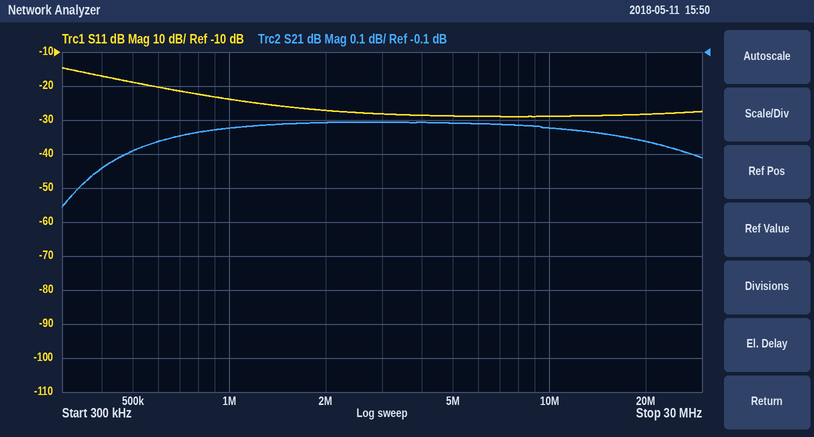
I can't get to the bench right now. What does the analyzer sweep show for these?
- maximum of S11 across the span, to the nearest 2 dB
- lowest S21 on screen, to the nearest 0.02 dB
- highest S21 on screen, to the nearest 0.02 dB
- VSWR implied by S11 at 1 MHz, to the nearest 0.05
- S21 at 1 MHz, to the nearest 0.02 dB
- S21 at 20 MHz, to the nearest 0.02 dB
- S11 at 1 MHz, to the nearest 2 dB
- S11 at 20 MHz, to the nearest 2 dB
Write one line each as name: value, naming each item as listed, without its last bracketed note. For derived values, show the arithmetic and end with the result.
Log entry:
maximum of S11 across the span, to the nearest 2 dB: -14 dB
lowest S21 on screen, to the nearest 0.02 dB: -0.56 dB
highest S21 on screen, to the nearest 0.02 dB: -0.30 dB
VSWR implied by S11 at 1 MHz, to the nearest 0.05: |Γ| = 10^(-24/20) = 0.0631; VSWR = (1 + 0.0631)/(1 − 0.0631) ≈ 1.13, so 1.15 to the nearest 0.05
S21 at 1 MHz, to the nearest 0.02 dB: -0.32 dB
S21 at 20 MHz, to the nearest 0.02 dB: -0.36 dB
S11 at 1 MHz, to the nearest 2 dB: -24 dB
S11 at 20 MHz, to the nearest 2 dB: -28 dB
